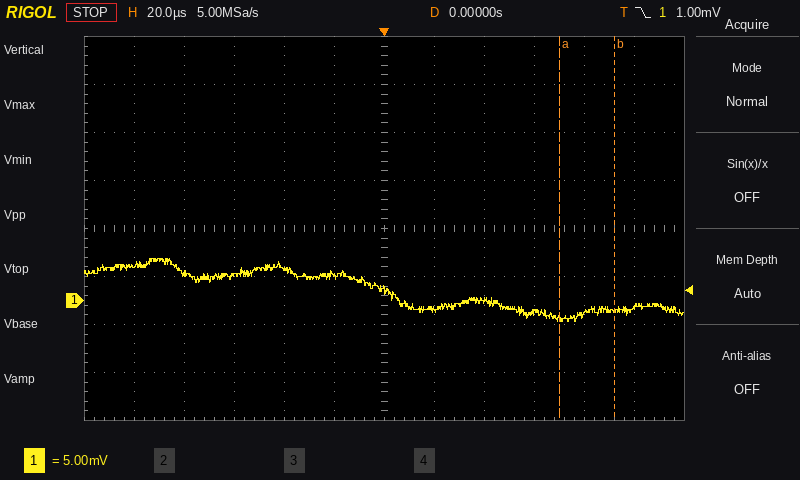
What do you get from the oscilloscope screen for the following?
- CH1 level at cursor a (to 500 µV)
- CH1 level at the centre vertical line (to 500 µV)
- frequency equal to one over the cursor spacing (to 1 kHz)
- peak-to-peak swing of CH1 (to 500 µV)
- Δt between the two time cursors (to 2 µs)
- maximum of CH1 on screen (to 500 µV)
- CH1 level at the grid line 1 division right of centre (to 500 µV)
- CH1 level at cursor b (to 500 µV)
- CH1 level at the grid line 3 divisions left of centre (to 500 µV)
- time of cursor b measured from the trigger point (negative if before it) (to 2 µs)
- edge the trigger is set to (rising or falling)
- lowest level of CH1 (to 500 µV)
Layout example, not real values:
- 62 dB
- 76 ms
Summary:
- -2.0 mV
- 1.0 mV
- 45 kHz
- 6.5 mV
- 22 µs
- 4.5 mV
- -1.0 mV
- -1.0 mV
- 2.5 mV
- +92 µs
- falling
- -2.0 mV
